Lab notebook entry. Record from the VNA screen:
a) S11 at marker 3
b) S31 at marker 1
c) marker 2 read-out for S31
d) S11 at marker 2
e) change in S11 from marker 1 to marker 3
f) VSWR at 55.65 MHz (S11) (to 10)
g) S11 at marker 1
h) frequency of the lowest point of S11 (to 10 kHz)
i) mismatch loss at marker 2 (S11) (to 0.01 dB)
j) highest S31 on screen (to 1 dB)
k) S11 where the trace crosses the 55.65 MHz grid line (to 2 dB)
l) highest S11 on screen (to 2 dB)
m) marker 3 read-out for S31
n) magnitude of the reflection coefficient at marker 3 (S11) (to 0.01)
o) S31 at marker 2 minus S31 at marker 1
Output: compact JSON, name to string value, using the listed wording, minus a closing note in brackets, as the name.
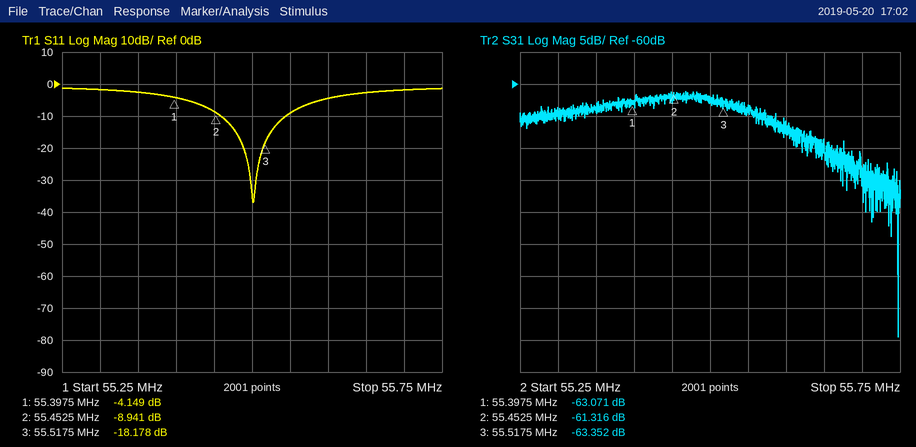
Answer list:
{"S11 at marker 3": "-18.178 dB", "S31 at marker 1": "-63.071 dB", "marker 2 read-out for S31": "-61.316 dB", "S11 at marker 2": "-8.941 dB", "change in S11 from marker 1 to marker 3": "-14.029 dB", "VSWR at 55.65 MHz (S11)": "10", "S11 at marker 1": "-4.149 dB", "frequency of the lowest point of S11": "55.50 MHz", "mismatch loss at marker 2 (S11)": "0.59 dB", "highest S31 on screen": "-61 dB", "S11 where the trace crosses the 55.65 MHz grid line": "-2 dB", "highest S11 on screen": "-2 dB", "marker 3 read-out for S31": "-63.352 dB", "magnitude of the reflection coefficient at marker 3 (S11)": "0.12", "S31 at marker 2 minus S31 at marker 1": "1.755 dB"}
